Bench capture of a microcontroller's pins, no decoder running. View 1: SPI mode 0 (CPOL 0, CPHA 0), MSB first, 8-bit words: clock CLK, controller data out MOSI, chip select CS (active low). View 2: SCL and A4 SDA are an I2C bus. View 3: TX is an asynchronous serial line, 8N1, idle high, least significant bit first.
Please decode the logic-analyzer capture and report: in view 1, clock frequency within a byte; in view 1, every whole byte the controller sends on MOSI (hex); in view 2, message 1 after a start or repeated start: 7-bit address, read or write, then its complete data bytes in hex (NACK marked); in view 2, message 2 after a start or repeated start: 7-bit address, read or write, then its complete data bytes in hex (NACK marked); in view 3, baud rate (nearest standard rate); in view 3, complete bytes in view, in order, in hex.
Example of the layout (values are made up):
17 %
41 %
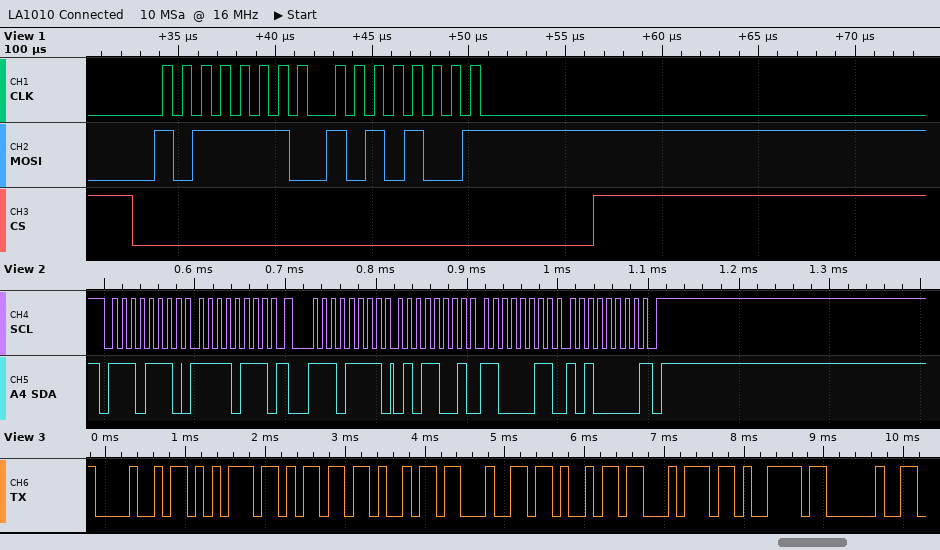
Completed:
1 MHz
0xBE 0xA9
0x77 write: F7
0x77 read: 59 C3 A0 NACK
9600 baud
0x48 0x75 0x6D 0x69 0x64 0x69 0x74 0x79 0x20
